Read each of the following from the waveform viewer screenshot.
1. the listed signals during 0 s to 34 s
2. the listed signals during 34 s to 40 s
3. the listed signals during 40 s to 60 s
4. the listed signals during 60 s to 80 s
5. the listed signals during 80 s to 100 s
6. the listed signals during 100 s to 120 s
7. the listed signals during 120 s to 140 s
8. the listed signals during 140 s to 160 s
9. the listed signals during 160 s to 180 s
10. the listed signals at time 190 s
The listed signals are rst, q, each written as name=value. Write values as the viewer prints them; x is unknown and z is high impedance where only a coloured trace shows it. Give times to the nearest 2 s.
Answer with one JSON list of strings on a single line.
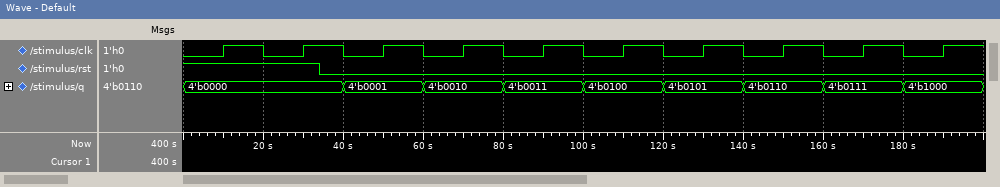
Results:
["rst=1, q=4'b0000", "rst=0, q=4'b0000", "rst=0, q=4'b0001", "rst=0, q=4'b0010", "rst=0, q=4'b0011", "rst=0, q=4'b0100", "rst=0, q=4'b0101", "rst=0, q=4'b0110", "rst=0, q=4'b0111", "rst=0, q=4'b1000"]
